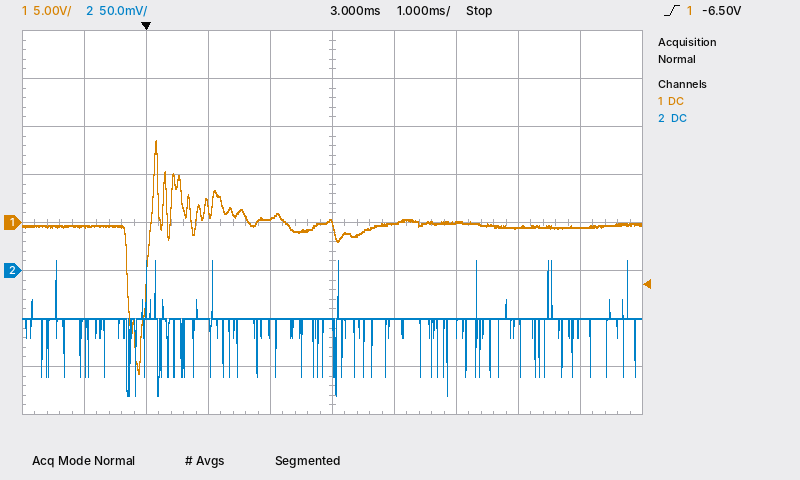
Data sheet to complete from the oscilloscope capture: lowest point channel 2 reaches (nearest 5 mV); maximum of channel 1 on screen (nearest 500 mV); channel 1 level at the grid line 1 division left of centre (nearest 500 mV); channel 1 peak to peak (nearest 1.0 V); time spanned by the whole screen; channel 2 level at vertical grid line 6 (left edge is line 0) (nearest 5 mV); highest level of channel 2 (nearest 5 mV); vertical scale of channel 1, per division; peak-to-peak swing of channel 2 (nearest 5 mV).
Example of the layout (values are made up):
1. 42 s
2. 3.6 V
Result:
1. -130 mV
2. 8.5 V
3. 500 mV
4. 24.0 V
5. 10 ms
6. -50 mV
7. 10 mV
8. 5 V
9. 140 mV
